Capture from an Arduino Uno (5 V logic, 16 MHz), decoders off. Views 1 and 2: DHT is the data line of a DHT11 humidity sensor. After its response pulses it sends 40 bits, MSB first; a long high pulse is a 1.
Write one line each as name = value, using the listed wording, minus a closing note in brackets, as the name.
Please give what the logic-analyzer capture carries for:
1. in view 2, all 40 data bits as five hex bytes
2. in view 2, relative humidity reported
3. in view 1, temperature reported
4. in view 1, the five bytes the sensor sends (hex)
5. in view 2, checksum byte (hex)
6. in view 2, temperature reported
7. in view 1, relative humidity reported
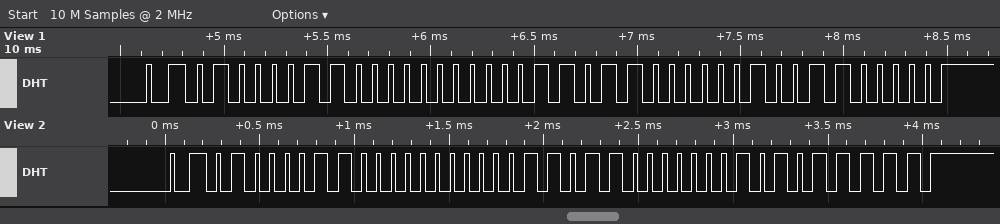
in view 2, all 40 data bits as five hex bytes = 43 00 1B 01 5F
in view 2, relative humidity reported = 67 %
in view 1, temperature reported = 27.2 °C
in view 1, the five bytes the sensor sends = 43 00 1B 02 60
in view 2, checksum byte = 0x5F
in view 2, temperature reported = 27.1 °C
in view 1, relative humidity reported = 67 %
